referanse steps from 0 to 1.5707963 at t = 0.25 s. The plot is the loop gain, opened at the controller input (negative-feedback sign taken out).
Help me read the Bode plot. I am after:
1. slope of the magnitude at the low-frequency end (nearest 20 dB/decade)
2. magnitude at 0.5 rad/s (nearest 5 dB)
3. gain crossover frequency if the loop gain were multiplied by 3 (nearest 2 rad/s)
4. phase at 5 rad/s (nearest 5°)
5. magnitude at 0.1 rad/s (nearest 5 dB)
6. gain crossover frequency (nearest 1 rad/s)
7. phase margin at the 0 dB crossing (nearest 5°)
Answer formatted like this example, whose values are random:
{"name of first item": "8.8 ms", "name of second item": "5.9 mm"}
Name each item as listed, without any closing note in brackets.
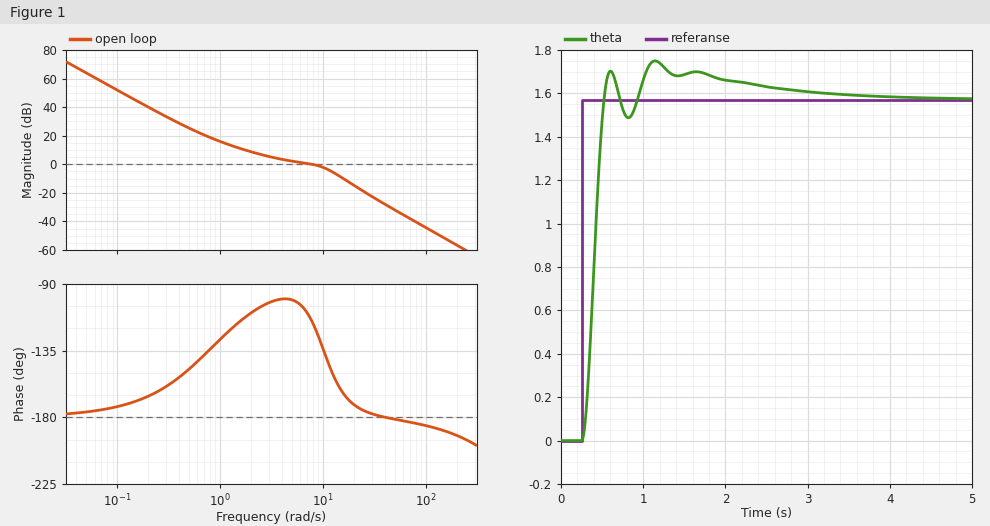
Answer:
{"slope of the magnitude at the low-frequency end": "-40 dB/decade", "magnitude at 0.5 rad/s": "25 dB", "gain crossover frequency if the loop gain were multiplied by 3": "16 rad/s", "phase at 5 rad/s": "-100°", "magnitude at 0.1 rad/s": "50 dB", "gain crossover frequency": "8 rad/s", "phase margin at the 0 dB crossing": "65°"}
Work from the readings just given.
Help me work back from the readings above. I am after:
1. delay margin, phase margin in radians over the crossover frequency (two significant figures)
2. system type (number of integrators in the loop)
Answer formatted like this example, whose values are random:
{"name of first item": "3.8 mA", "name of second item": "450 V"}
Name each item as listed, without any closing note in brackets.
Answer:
{"delay margin, phase margin in radians over the crossover frequency": "0.14 s", "system type": "2"}
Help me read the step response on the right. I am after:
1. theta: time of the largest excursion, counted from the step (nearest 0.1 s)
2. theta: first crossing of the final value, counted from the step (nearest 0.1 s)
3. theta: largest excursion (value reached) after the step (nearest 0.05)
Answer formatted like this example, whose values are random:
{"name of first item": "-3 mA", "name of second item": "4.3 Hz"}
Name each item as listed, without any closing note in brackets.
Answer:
{"theta: time of the largest excursion, counted from the step": "0.9 s", "theta: first crossing of the final value, counted from the step": "0.3 s", "theta: largest excursion (value reached) after the step": "1.75"}
